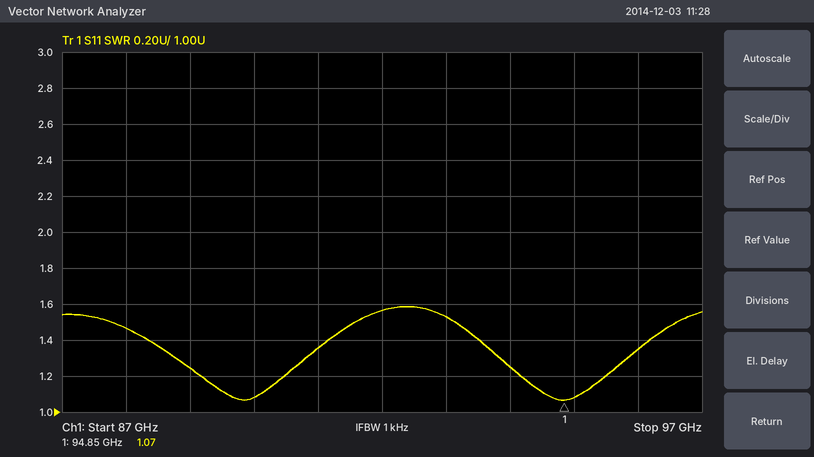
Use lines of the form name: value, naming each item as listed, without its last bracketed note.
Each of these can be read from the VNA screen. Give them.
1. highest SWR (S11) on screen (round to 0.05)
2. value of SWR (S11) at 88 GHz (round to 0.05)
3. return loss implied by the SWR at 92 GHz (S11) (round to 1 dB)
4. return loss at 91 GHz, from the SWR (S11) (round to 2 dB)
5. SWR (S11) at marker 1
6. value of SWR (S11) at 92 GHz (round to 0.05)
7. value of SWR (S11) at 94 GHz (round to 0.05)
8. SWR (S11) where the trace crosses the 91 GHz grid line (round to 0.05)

highest SWR (S11) on screen: 1.60
value of SWR (S11) at 88 GHz: 1.45
return loss implied by the SWR at 92 GHz (S11): 13 dB
return loss at 91 GHz, from the SWR (S11): 16 dB
SWR (S11) at marker 1: 1.07
value of SWR (S11) at 92 GHz: 1.55
value of SWR (S11) at 94 GHz: 1.25
SWR (S11) where the trace crosses the 91 GHz grid line: 1.35
